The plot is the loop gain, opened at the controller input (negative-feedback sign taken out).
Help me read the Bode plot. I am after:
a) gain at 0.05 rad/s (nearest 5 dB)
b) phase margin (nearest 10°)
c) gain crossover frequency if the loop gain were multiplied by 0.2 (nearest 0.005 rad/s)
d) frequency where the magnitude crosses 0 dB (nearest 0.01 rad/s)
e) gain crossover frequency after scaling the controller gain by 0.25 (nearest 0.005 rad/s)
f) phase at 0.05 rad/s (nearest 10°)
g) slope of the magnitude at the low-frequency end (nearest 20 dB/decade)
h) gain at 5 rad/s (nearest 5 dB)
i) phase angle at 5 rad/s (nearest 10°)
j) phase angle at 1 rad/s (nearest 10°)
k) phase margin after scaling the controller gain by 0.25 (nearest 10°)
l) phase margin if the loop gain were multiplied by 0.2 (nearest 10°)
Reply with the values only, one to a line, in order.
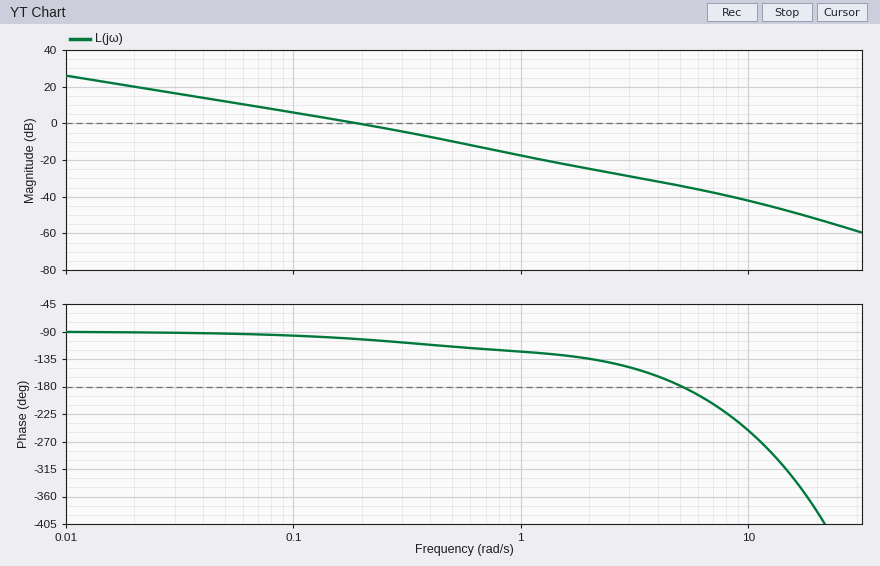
10 dB
80°
0.040 rad/s
0.19 rad/s
0.050 rad/s
-90°
-20 dB/decade
-35 dB
-180°
-120°
90°
90°
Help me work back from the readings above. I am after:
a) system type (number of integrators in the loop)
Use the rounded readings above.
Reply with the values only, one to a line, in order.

1
